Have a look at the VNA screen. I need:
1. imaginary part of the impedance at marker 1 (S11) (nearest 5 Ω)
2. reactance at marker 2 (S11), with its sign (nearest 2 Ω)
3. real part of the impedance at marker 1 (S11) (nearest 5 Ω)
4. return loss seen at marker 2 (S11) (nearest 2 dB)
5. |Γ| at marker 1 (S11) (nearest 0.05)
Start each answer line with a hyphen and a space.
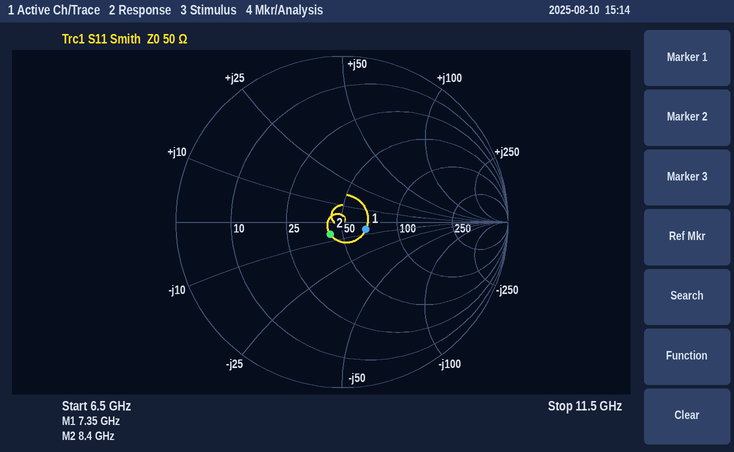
- -5 Ω
- -6 Ω
- 65 Ω
- 20 dB
- 0.15
